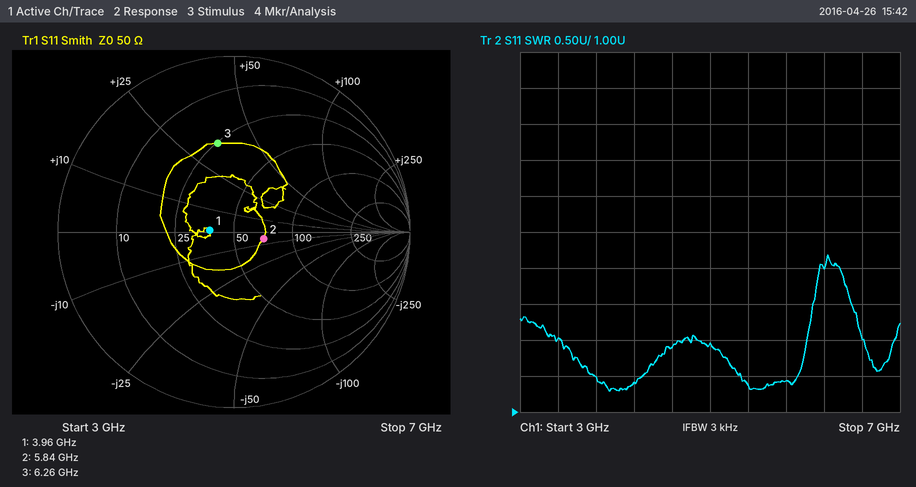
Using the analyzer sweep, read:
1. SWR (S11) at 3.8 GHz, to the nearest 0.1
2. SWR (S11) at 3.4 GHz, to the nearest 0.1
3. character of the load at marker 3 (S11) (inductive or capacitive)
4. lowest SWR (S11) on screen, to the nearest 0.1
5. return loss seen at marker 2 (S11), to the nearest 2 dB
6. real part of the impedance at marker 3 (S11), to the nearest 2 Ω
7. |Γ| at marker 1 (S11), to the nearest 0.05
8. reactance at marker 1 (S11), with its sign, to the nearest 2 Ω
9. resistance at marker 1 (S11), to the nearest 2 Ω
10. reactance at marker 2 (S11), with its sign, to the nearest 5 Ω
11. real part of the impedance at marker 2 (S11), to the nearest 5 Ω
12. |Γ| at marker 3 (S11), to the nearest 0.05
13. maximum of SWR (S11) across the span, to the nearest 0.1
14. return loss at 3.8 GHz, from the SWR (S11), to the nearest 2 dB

1.5
2.0
inductive
1.3
16 dB
26 Ω
0.15
0 Ω
38 Ω
-5 Ω
70 Ω
0.50
3.2
14 dB
